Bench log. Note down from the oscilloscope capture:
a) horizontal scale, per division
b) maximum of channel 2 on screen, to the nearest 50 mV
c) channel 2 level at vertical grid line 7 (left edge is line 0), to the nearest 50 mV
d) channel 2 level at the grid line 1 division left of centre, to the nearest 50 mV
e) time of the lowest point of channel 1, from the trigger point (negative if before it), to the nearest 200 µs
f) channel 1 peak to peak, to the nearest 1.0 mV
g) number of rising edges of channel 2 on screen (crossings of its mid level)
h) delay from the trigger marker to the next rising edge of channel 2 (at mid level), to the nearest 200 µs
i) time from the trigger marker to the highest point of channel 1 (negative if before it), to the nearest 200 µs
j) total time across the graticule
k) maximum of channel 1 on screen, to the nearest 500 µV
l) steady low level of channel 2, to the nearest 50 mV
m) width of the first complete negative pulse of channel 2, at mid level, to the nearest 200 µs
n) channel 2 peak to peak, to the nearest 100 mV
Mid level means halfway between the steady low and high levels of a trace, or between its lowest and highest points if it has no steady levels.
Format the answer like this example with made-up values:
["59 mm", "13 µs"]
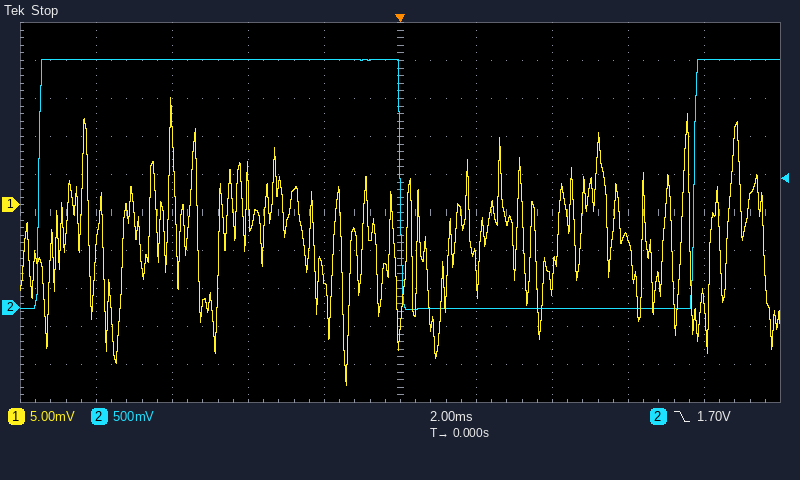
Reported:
["2 ms", "3.25 V", "0 mV", "3.25 V", "-1.4 ms", "38.0 mV", "2", "7.8 ms", "-6.0 ms", "20 ms", "14.0 mV", "0 mV", "7.8 ms", "3.30 V"]
